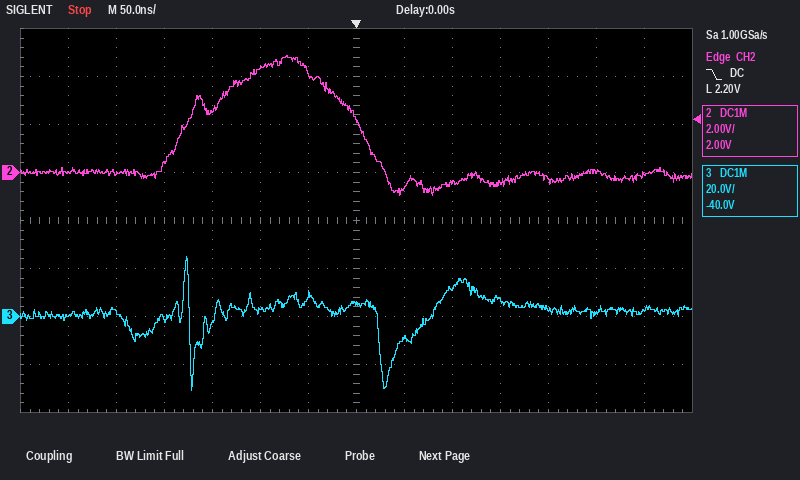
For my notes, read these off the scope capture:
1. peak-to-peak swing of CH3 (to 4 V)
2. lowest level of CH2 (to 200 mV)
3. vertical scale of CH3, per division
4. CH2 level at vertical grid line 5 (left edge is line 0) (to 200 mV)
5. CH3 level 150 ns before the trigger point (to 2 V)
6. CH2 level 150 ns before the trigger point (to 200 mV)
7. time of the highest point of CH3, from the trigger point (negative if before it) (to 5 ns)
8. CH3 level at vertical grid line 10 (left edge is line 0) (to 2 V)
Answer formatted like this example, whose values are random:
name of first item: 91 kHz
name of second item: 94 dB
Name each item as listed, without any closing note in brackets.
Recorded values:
peak-to-peak swing of CH3: 56 V
lowest level of CH2: -1.0 V
vertical scale of CH3, per division: 20 V
CH2 level at vertical grid line 5 (left edge is line 0): 4.4 V
CH3 level 150 ns before the trigger point: -4 V
CH2 level 150 ns before the trigger point: 2.6 V
time of the highest point of CH3, from the trigger point (negative if before it): -175 ns
CH3 level at vertical grid line 10 (left edge is line 0): 6 V
